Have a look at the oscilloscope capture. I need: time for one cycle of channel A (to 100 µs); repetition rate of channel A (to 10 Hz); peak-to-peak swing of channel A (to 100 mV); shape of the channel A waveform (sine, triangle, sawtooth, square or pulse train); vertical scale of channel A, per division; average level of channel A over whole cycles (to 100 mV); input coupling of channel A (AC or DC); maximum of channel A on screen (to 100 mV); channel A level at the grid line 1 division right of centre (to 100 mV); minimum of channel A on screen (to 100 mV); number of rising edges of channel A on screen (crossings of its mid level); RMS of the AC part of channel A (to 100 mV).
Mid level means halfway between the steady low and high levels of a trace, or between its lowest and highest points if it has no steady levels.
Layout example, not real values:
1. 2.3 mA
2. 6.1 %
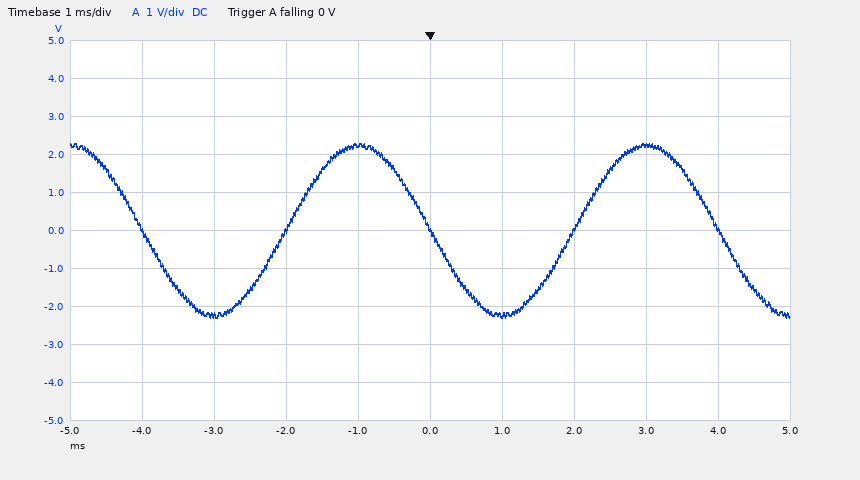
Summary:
1. 4.0 ms
2. 250 Hz
3. 4.6 V
4. sine
5. 1 V
6. 0.0 V
7. DC
8. 2.3 V
9. -2.2 V
10. -2.3 V
11. 2
12. 1.6 V
